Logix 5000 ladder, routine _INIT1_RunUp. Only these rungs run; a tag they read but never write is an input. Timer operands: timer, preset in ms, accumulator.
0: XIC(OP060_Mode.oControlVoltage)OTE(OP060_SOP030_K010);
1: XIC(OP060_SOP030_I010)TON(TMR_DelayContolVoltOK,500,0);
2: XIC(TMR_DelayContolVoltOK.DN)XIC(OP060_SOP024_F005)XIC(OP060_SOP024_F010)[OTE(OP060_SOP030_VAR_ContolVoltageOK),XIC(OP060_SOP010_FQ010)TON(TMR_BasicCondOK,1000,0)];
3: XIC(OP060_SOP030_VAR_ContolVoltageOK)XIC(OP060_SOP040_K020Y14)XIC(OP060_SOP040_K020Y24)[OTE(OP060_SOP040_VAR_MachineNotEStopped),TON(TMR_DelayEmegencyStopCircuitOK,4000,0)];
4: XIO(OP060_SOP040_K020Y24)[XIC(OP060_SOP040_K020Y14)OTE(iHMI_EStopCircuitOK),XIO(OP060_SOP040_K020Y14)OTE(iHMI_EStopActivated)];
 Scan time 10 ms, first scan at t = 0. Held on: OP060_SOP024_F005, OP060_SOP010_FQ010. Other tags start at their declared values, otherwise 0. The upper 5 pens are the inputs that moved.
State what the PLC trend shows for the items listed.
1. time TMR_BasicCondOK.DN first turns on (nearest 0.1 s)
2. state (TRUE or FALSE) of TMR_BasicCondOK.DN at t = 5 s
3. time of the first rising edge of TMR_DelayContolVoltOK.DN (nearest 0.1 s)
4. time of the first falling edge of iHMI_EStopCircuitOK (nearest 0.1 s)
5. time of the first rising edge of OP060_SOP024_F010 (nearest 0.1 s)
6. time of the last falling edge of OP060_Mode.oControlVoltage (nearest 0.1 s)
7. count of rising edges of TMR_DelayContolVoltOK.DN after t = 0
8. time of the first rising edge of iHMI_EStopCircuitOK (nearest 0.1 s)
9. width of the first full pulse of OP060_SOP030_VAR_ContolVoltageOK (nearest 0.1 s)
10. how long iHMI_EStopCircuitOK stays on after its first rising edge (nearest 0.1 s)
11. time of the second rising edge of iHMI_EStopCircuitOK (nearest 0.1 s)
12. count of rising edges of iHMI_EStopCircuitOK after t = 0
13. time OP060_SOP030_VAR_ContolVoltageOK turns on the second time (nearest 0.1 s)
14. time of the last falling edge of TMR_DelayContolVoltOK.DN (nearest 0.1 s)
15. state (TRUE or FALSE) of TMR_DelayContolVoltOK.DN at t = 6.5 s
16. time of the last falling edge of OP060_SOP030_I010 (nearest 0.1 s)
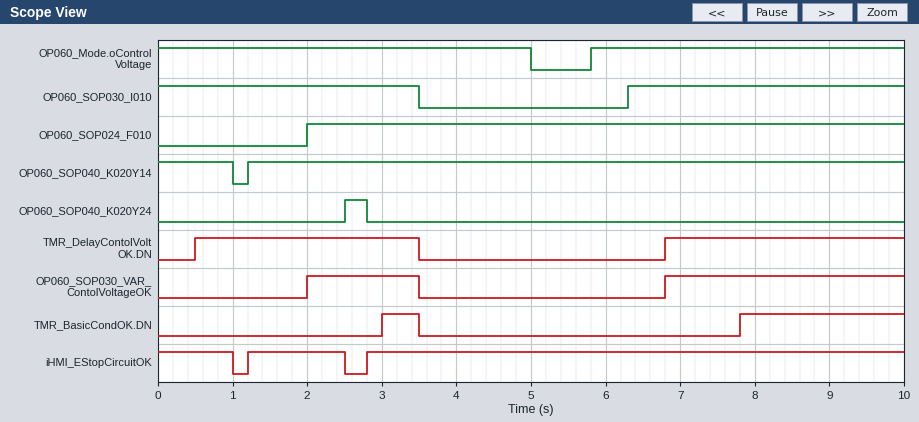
3.0 s
FALSE
0.5 s
1.0 s
2.0 s
5.0 s
2
1.2 s
1.5 s
1.3 s
2.8 s
2
6.8 s
3.5 s
FALSE
3.5 s
